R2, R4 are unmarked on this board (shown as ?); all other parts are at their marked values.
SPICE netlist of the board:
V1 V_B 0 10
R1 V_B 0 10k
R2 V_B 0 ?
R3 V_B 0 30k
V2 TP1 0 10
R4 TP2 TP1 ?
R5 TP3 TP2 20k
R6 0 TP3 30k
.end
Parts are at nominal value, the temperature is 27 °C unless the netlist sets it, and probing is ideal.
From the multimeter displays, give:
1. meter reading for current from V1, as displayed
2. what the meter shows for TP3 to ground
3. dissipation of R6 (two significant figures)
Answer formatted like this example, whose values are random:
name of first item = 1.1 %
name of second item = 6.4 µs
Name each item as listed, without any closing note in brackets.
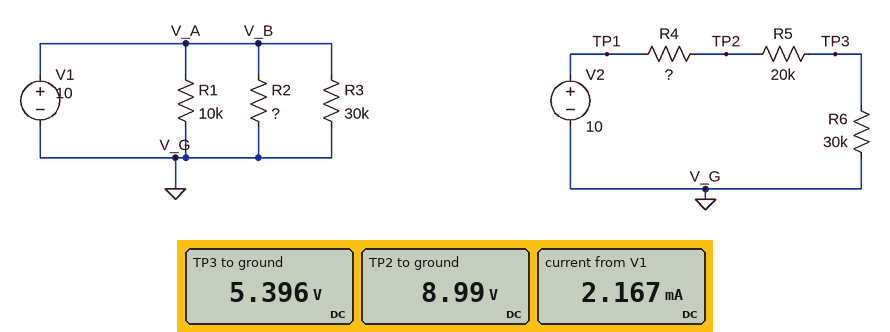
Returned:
meter reading for current from V1, as displayed = 2.167 mA
what the meter shows for TP3 to ground = 5.396 V
dissipation of R6 = 970 µW
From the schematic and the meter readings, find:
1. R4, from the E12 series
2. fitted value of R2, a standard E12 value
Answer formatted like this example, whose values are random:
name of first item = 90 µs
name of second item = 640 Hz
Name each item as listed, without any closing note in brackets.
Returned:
R4, from the E12 series = 5.6 kΩ
fitted value of R2, a standard E12 value = 12 kΩ
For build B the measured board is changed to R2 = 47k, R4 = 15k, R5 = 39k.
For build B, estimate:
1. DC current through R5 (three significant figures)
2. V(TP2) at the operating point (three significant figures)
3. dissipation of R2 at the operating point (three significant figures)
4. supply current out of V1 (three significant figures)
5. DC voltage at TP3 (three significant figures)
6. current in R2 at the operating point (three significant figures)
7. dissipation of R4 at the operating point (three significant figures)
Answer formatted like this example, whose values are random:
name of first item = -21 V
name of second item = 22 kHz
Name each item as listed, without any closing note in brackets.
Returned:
DC current through R5 = 119 µA
V(TP2) at the operating point = 8.21 V
dissipation of R2 at the operating point = 2.13 mW
supply current out of V1 = 1.55 mA
DC voltage at TP3 = 3.57 V
current in R2 at the operating point = 213 µA
dissipation of R4 at the operating point = 213 µW
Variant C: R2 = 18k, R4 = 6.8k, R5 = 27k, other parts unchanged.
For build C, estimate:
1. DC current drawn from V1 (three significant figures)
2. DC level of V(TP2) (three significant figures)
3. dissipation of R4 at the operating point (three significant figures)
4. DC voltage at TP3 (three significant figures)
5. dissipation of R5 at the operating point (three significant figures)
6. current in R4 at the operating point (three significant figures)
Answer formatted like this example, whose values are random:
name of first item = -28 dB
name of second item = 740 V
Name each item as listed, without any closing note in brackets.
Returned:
DC current drawn from V1 = 1.89 mA
DC level of V(TP2) = 8.93 V
dissipation of R4 at the operating point = 167 µW
DC voltage at TP3 = 4.70 V
dissipation of R5 at the operating point = 663 µW
current in R4 at the operating point = 157 µA
